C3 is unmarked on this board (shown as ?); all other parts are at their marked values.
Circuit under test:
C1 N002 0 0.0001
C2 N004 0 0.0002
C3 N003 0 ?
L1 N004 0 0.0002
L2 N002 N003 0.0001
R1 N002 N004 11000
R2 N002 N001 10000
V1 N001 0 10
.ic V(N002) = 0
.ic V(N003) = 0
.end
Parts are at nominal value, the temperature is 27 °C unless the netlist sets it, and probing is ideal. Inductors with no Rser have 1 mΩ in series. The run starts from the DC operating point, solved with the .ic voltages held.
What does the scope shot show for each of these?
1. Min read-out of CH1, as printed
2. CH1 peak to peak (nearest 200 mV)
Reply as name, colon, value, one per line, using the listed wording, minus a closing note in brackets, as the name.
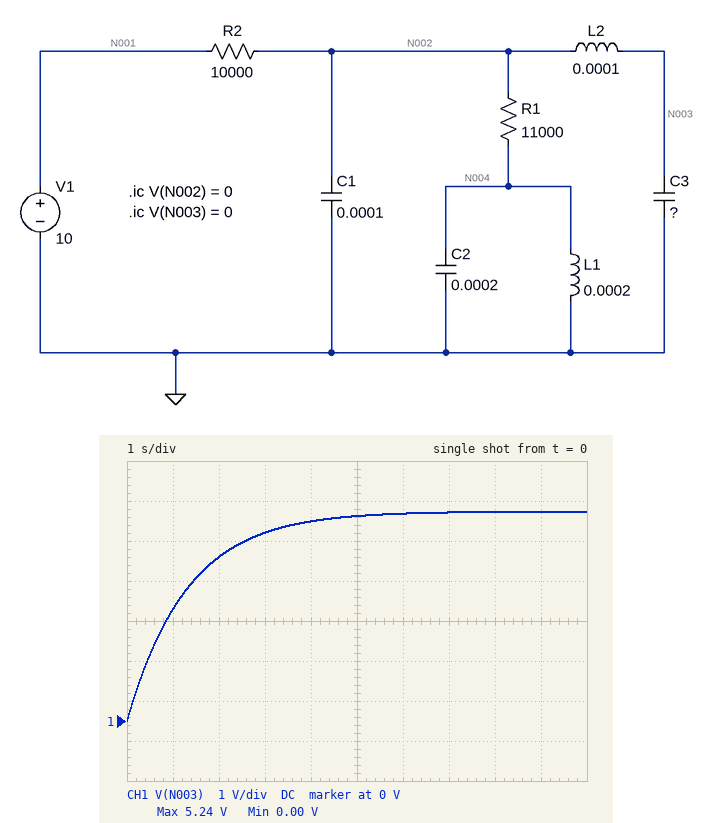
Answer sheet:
Min read-out of CH1, as printed: 0.00 V
CH1 peak to peak: 5.2 V
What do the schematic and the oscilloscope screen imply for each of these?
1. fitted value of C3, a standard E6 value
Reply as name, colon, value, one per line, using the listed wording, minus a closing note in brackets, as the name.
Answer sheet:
fitted value of C3, a standard E6 value: 150 µF
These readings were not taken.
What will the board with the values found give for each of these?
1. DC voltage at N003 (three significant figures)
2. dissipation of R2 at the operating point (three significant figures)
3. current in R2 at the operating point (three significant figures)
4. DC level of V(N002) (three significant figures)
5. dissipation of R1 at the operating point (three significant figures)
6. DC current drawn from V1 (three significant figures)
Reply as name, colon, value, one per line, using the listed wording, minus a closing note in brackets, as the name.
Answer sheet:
DC voltage at N003: 5.24 V
dissipation of R2 at the operating point: 2.27 mW
current in R2 at the operating point: 476 µA
DC level of V(N002): 5.24 V
dissipation of R1 at the operating point: 2.49 mW
DC current drawn from V1: 476 µA
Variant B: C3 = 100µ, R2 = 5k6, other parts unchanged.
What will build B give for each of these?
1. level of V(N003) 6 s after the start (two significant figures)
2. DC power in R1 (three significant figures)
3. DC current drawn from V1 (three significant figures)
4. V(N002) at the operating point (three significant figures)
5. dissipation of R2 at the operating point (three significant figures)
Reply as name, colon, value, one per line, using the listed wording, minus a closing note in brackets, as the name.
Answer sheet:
level of V(N003) 6 s after the start: 6.6 V
DC power in R1: 3.99 mW
DC current drawn from V1: 602 µA
V(N002) at the operating point: 6.63 V
dissipation of R2 at the operating point: 2.03 mW
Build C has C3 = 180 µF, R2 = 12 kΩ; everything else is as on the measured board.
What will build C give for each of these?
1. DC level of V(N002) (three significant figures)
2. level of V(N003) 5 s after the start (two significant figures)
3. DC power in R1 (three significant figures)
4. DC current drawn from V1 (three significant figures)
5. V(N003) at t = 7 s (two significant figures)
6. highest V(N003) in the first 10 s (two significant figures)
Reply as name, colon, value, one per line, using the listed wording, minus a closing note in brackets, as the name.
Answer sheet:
DC level of V(N002): 4.78 V
level of V(N003) 5 s after the start: 4.6 V
DC power in R1: 2.08 mW
DC current drawn from V1: 435 µA
V(N003) at t = 7 s: 4.7 V
highest V(N003) in the first 10 s: 4.8 V
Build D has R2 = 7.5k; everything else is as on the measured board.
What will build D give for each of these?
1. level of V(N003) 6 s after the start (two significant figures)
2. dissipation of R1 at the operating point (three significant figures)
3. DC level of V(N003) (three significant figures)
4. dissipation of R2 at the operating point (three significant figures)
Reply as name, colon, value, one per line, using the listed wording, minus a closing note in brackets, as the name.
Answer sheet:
level of V(N003) 6 s after the start: 5.9 V
dissipation of R1 at the operating point: 3.21 mW
DC level of V(N003): 5.95 V
dissipation of R2 at the operating point: 2.19 mW
